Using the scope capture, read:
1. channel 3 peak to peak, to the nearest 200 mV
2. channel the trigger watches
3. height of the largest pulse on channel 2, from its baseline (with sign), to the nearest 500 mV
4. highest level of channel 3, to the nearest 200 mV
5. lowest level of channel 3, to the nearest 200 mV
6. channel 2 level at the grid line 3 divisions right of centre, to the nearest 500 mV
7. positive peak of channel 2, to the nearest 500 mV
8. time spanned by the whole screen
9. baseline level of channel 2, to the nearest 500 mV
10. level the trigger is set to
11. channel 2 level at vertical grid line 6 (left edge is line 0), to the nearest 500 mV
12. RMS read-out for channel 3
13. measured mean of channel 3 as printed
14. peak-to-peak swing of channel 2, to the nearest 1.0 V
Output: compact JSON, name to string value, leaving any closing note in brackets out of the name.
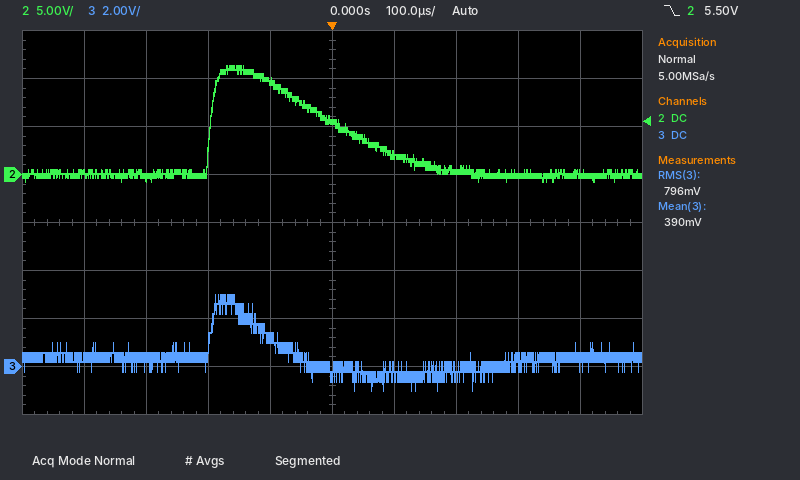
{"channel 3 peak to peak, to the nearest 200 mV": "4.0 V", "channel the trigger watches": "channel 2", "height of the largest pulse on channel 2, from its baseline (with sign), to the nearest 500 mV": "+11.5 V", "highest level of channel 3, to the nearest 200 mV": "3.0 V", "lowest level of channel 3, to the nearest 200 mV": "-1.0 V", "channel 2 level at the grid line 3 divisions right of centre, to the nearest 500 mV": "0.0 V", "positive peak of channel 2, to the nearest 500 mV": "11.5 V", "time spanned by the whole screen": "1 ms", "baseline level of channel 2, to the nearest 500 mV": "0.0 V", "level the trigger is set to": "5.50 V", "channel 2 level at vertical grid line 6 (left edge is line 0), to the nearest 500 mV": "2.0 V", "RMS read-out for channel 3": "796 mV", "measured mean of channel 3 as printed": "390 mV", "peak-to-peak swing of channel 2, to the nearest 1.0 V": "12.0 V"}
